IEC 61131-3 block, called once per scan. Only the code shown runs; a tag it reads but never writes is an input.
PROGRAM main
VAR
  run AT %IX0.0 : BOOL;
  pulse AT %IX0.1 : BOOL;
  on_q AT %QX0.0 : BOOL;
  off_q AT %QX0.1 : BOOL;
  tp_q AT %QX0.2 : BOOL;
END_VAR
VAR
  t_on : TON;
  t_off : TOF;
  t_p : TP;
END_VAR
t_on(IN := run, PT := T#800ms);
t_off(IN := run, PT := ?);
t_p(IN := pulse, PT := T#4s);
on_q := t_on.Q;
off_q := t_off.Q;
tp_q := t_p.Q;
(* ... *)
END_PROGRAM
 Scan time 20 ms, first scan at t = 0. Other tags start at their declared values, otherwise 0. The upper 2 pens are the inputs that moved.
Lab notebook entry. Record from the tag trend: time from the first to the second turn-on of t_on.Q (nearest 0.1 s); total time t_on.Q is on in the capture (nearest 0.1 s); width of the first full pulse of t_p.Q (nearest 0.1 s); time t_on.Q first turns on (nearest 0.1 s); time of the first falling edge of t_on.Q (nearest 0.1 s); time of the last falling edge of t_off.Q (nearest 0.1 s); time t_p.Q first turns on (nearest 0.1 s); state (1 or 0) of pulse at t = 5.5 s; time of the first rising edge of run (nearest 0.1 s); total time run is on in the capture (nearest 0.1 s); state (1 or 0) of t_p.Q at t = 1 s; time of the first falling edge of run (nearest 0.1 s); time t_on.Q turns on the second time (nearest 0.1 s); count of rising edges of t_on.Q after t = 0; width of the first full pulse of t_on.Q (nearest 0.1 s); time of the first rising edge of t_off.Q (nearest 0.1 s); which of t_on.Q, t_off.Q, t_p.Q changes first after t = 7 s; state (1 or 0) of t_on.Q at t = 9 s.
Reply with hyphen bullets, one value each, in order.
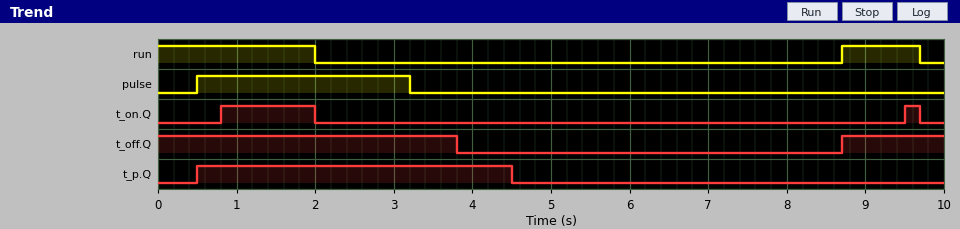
- 8.7 s
- 1.4 s
- 4.0 s
- 0.8 s
- 2.0 s
- 3.8 s
- 0.5 s
- 0
- 8.7 s
- 3.0 s
- 1
- 2.0 s
- 9.5 s
- 2
- 1.2 s
- 8.7 s
- t_off.Q
- 0
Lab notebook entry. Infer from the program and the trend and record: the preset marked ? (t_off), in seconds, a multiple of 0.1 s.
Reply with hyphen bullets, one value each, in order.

- 1.8 s
